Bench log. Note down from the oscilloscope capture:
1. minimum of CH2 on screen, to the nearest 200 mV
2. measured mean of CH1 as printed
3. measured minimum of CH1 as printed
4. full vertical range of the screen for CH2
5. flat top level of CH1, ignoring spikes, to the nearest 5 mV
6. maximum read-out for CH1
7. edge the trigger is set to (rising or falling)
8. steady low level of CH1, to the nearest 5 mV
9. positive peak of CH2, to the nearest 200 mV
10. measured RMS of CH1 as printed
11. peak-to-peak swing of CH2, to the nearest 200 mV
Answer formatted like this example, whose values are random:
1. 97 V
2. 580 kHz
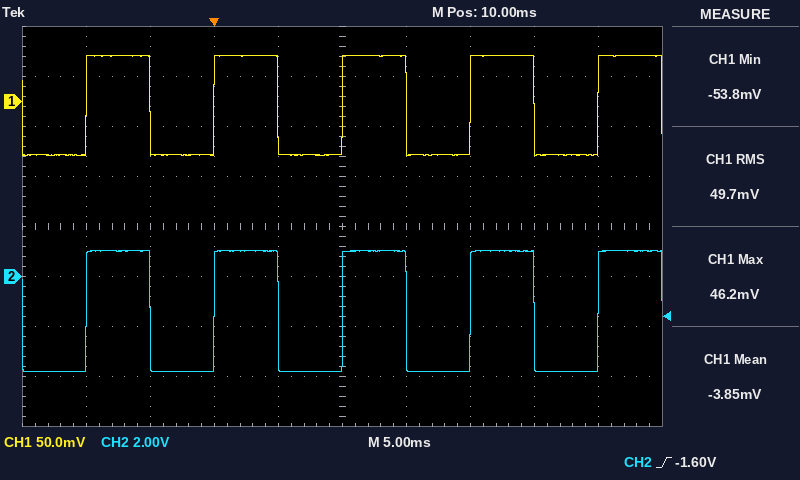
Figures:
1. -3.8 V
2. -3.85 mV
3. -53.8 mV
4. 16 V
5. 45 mV
6. 46.2 mV
7. rising
8. -55 mV
9. 1.0 V
10. 49.7 mV
11. 4.8 V
